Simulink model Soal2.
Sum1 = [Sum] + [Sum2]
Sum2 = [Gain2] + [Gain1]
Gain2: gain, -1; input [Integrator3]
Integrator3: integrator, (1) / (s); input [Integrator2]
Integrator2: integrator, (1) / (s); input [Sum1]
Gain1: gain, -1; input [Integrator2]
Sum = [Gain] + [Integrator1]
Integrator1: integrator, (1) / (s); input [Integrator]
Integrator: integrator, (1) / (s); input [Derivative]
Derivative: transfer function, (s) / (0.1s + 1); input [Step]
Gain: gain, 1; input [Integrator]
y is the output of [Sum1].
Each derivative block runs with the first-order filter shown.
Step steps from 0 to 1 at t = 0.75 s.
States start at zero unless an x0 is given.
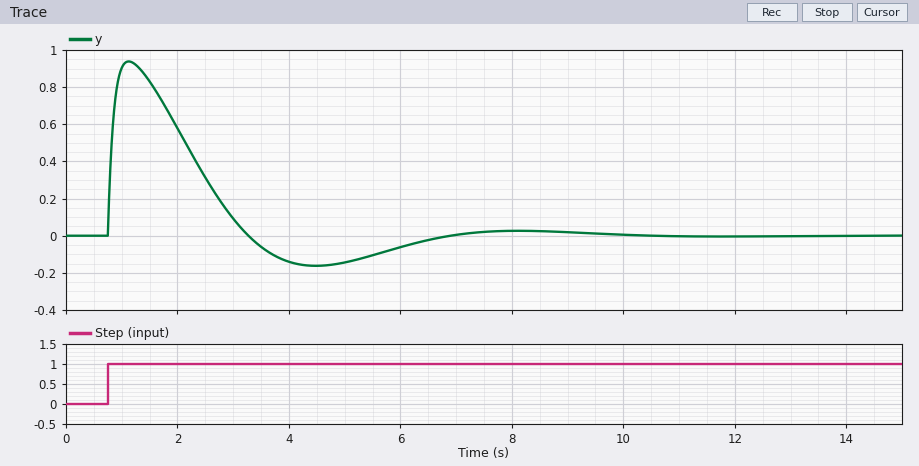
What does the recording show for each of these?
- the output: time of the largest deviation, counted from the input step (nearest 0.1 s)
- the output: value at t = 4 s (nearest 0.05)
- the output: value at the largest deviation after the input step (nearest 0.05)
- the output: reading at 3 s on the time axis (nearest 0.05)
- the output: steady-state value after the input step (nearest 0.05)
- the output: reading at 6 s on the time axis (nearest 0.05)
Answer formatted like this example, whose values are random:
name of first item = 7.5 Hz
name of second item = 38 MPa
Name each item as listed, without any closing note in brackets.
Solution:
the output: time of the largest deviation, counted from the input step = 0.4 s
the output: value at t = 4 s = -0.15
the output: value at the largest deviation after the input step = 0.95
the output: reading at 3 s on the time axis = 0.10
the output: steady-state value after the input step = 0.00
the output: reading at 6 s on the time axis = -0.05
